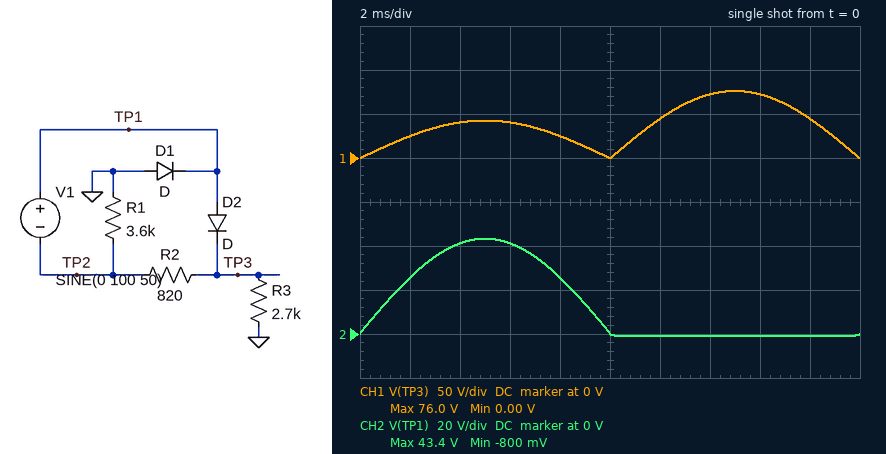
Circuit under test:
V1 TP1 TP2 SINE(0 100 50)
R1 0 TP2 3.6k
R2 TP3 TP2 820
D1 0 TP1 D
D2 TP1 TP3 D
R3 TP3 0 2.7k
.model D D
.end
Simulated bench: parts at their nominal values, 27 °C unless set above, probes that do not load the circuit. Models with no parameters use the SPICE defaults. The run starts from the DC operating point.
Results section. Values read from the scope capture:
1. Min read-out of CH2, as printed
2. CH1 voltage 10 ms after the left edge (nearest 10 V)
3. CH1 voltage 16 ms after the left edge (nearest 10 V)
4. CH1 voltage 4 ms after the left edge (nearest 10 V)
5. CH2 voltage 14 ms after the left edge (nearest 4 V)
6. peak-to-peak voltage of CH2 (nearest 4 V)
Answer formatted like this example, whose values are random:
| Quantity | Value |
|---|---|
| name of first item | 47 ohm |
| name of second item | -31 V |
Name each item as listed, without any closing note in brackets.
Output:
| Quantity | Value |
|---|---|
| Min read-out of CH2, as printed | -800 mV |
| CH1 voltage 10 ms after the left edge | 0 V |
| CH1 voltage 16 ms after the left edge | 70 V |
| CH1 voltage 4 ms after the left edge | 40 V |
| CH2 voltage 14 ms after the left edge | 0 V |
| peak-to-peak voltage of CH2 | 44 V |
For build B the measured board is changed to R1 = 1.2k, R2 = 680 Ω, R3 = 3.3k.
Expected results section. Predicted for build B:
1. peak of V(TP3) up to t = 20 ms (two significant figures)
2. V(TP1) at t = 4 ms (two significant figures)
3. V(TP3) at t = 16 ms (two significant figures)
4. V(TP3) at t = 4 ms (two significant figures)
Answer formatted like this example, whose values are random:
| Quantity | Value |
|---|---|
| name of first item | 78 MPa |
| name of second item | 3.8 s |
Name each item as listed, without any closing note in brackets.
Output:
| Quantity | Value |
|---|---|
| peak of V(TP3) up to t = 20 ms | 82 V |
| V(TP1) at t = 4 ms | 70 V |
| V(TP3) at t = 16 ms | 78 V |
| V(TP3) at t = 4 ms | 69 V |
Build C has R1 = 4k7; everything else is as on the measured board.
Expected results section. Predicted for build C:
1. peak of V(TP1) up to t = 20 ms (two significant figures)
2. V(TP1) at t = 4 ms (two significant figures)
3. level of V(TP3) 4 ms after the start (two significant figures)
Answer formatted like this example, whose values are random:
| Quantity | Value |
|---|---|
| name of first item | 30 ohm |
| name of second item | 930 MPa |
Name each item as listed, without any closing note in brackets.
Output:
| Quantity | Value |
|---|---|
| peak of V(TP1) up to t = 20 ms | 37 V |
| V(TP1) at t = 4 ms | 35 V |
| level of V(TP3) 4 ms after the start | 34 V |
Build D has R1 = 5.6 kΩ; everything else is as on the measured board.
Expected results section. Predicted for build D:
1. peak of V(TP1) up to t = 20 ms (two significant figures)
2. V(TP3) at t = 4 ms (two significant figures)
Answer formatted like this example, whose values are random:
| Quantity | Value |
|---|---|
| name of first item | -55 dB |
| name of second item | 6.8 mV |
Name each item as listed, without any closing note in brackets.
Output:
| Quantity | Value |
|---|---|
| peak of V(TP1) up to t = 20 ms | 33 V |
| V(TP3) at t = 4 ms | 31 V |
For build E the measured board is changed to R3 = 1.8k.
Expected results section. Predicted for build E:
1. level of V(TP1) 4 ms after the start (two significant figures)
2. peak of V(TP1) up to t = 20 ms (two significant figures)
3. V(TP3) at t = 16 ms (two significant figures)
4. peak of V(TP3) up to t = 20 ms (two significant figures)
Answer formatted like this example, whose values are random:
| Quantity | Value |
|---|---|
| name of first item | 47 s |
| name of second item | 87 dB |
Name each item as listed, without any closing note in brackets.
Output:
| Quantity | Value |
|---|---|
| level of V(TP1) 4 ms after the start | 32 V |
| peak of V(TP1) up to t = 20 ms | 34 V |
| V(TP3) at t = 16 ms | 65 V |
| peak of V(TP3) up to t = 20 ms | 68 V |
